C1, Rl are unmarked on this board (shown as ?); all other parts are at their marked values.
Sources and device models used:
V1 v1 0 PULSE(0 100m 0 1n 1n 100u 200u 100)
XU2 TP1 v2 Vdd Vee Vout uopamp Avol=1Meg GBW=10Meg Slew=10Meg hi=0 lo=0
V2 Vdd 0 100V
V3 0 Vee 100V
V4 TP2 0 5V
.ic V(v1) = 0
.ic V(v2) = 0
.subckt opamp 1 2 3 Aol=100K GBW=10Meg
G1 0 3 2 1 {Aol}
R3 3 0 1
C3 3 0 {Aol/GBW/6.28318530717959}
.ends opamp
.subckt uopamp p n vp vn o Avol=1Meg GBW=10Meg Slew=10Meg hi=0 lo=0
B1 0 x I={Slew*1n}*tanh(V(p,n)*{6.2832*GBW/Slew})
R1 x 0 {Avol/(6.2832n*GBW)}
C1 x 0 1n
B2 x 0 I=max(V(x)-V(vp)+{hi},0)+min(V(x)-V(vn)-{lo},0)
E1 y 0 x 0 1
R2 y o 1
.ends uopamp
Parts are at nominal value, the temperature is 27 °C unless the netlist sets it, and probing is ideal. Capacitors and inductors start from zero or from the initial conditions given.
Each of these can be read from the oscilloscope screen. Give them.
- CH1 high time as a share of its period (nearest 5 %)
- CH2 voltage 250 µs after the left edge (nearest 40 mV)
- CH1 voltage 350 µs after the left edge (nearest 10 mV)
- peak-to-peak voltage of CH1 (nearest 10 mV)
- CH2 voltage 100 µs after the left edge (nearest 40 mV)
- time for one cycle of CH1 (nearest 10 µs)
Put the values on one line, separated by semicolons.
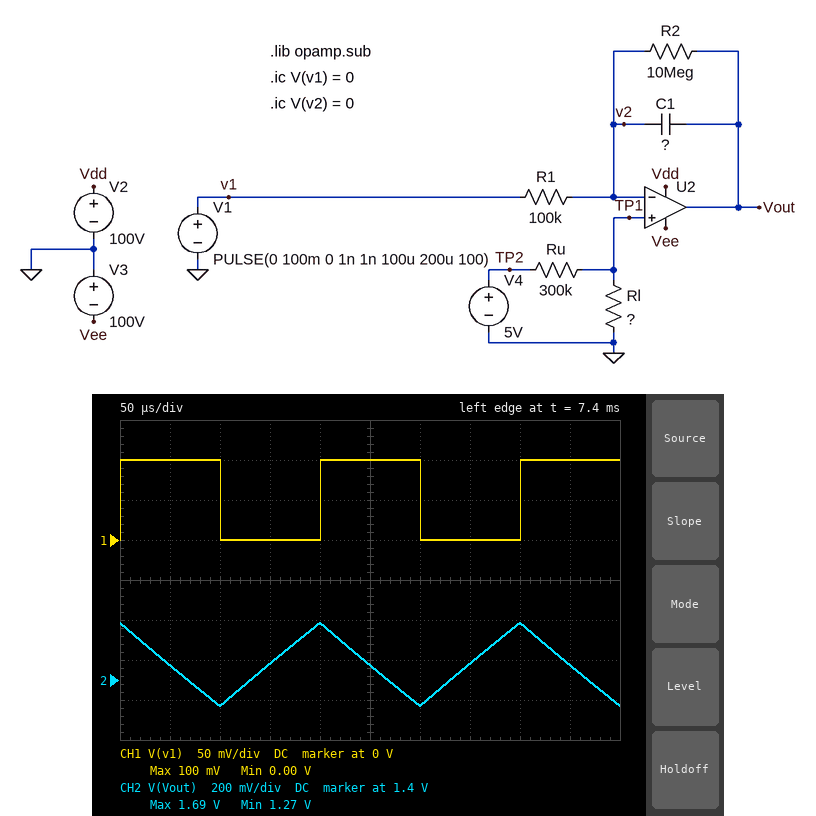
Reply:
50 %; 1.48 V; 0 V; 100 mV; 1.28 V; 200 µs
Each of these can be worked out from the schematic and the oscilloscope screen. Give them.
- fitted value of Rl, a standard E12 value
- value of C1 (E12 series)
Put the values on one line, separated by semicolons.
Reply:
3.9 kΩ; 120 pF
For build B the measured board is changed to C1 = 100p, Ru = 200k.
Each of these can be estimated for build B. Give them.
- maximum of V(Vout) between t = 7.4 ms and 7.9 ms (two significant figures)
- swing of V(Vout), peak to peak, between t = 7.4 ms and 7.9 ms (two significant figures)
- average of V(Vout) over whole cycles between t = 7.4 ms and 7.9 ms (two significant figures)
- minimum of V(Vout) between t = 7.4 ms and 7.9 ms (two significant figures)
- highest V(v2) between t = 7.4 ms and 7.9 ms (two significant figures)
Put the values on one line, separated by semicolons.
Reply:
4.9 V; 500 mV; 4.7 V; 4.4 V; 96 mV
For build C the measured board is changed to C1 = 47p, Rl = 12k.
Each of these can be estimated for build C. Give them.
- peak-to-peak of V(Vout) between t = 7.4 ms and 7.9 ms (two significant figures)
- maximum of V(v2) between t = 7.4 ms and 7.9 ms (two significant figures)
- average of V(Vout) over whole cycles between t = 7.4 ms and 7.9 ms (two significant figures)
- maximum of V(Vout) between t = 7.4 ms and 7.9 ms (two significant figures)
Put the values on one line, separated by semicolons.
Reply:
1.1 V; 190 mV; 14 V; 15 V
